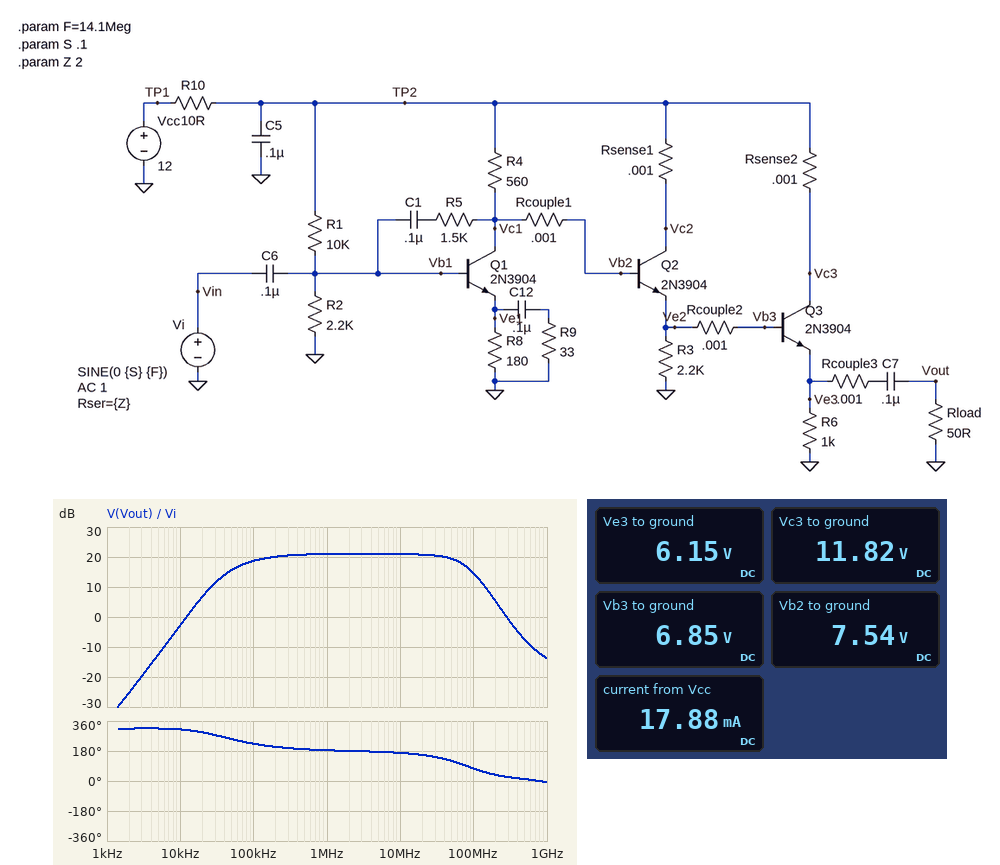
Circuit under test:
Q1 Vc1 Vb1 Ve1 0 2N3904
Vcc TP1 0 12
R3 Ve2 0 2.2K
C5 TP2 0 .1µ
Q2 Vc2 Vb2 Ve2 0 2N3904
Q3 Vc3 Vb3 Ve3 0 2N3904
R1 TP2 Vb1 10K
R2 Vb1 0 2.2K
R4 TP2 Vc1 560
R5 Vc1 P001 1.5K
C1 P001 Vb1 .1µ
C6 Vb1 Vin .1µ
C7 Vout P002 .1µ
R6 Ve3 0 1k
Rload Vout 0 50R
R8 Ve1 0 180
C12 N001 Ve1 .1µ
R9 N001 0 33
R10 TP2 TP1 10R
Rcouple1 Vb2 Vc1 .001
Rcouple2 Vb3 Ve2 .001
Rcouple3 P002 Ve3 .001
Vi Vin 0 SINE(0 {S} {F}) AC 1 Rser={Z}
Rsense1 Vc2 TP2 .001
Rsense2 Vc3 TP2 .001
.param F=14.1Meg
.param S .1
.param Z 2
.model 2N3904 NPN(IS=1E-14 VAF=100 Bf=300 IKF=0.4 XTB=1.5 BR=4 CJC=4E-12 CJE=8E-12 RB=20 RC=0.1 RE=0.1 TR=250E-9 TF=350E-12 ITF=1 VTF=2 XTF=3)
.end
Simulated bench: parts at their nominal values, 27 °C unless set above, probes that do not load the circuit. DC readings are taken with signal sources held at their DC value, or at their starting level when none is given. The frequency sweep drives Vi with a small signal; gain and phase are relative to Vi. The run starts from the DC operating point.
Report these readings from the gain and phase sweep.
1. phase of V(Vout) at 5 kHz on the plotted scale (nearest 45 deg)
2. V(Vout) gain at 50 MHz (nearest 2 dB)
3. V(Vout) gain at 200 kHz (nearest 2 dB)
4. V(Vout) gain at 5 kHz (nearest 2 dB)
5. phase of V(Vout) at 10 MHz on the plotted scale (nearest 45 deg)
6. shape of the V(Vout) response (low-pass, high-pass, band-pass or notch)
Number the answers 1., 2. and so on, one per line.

1. 315 deg
2. 20 dB
3. 20 dB
4. -12 dB
5. 180 deg
6. band-pass
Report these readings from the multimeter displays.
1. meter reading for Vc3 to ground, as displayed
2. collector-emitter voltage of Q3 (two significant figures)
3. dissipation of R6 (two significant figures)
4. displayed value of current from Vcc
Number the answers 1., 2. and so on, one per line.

1. 11.82 V
2. 5.7 V
3. 38 mW
4. 17.88 mA
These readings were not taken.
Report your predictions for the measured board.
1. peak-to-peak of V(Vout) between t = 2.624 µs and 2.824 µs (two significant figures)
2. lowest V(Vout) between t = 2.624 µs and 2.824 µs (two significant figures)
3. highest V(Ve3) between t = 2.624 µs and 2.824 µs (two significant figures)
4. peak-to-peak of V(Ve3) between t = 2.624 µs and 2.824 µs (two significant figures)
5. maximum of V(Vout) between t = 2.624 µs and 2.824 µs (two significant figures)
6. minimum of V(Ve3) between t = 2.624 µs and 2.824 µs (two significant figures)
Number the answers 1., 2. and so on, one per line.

1. 1.4 V
2. -350 mV
3. 7.3 V
4. 1.4 V
5. 1.0 V
6. 5.9 V
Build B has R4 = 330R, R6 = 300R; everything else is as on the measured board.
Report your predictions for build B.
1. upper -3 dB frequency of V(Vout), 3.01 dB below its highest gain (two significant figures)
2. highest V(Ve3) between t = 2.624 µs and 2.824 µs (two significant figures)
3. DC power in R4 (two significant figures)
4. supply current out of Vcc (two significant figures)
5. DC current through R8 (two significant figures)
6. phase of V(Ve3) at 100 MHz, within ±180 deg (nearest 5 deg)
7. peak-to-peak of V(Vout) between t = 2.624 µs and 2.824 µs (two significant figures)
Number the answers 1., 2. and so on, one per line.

1. 89 MHz
2. 8.5 V
3. 18 mW
4. 38 mA
5. 7.5 mA
6. 85 deg
7. 1.6 V
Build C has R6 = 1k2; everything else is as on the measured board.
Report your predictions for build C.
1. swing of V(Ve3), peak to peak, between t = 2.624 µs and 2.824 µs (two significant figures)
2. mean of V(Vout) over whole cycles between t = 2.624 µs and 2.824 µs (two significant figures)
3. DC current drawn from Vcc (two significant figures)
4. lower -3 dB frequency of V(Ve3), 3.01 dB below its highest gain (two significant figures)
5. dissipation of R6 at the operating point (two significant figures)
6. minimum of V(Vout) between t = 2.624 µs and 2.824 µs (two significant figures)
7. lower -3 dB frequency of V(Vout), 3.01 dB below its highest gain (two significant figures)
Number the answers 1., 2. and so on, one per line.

1. 1.3 V
2. 180 mV
3. 17 mA
4. 63 kHz
5. 32 mW
6. -300 mV
7. 79 kHz
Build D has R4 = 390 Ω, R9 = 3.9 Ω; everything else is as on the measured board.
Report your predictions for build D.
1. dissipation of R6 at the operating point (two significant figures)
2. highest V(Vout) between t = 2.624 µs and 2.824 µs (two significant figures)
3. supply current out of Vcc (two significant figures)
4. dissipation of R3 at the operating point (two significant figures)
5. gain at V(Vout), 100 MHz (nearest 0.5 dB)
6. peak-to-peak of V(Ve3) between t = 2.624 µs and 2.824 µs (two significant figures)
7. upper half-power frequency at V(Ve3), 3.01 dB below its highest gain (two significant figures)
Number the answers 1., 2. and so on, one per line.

1. 55 mW
2. 1.8 V
3. 20 mA
4. 30 mW
5. 22.5 dB
6. 2.3 V
7. 45 MHz
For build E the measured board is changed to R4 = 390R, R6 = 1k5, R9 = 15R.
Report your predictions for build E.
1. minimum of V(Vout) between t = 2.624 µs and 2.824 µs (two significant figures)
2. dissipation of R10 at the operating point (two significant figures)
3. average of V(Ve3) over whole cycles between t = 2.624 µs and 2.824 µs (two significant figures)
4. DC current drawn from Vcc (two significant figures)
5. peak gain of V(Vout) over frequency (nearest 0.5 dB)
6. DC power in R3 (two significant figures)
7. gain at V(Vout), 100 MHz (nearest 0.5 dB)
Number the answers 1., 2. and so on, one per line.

1. -320 mV
2. 3.0 mW
3. 7.9 V
4. 17 mA
5. 23.5 dB
6. 30 mW
7. 18.0 dB
